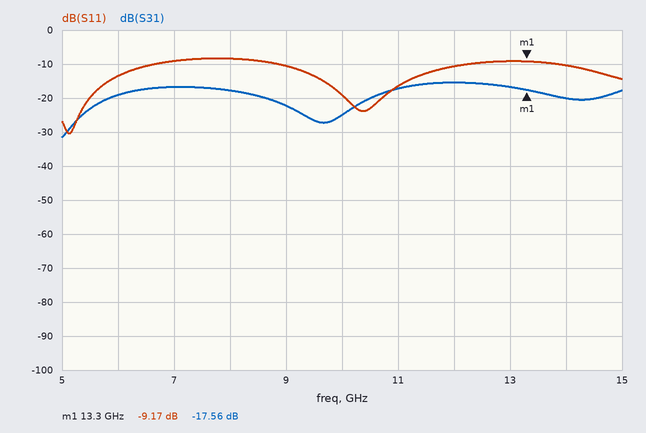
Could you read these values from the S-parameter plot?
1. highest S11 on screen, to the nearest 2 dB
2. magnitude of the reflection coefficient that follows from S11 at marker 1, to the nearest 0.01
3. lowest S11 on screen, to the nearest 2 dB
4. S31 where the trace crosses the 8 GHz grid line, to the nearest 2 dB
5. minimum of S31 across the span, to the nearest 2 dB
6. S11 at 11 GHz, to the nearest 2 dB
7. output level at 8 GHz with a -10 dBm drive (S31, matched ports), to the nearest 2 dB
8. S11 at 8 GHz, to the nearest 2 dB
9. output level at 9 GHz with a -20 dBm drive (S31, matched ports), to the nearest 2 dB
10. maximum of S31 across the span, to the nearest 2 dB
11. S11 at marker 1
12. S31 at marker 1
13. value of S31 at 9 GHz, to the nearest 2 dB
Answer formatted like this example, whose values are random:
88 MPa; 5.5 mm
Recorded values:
-8 dB; 0.35; -30 dB; -18 dB; -32 dB; -16 dB; -28 dBm; -8 dB; -42 dBm; -16 dB; -9.17 dB; -17.56 dB; -22 dB
